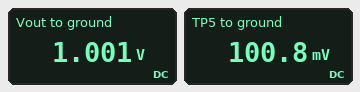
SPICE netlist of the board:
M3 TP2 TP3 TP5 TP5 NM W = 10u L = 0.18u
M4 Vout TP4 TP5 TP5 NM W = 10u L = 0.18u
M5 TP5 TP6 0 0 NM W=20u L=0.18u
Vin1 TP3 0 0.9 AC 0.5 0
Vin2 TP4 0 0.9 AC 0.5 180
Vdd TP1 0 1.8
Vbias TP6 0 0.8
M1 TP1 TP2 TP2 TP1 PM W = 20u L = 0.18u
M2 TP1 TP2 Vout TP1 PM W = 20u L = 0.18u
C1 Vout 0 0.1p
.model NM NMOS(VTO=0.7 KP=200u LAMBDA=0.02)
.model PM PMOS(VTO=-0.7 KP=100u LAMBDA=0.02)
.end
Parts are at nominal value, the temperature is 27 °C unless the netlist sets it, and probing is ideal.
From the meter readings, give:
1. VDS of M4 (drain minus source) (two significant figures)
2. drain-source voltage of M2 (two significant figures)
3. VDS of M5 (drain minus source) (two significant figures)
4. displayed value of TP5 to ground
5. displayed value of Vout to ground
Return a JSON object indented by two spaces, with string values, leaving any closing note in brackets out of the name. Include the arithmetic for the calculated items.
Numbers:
{
  "VDS of M4 (drain minus source)": "1.001 V - 100.8 mV = 900 mV",
  "drain-source voltage of M2": "1.8 V - 1.001 V = 800 mV",
  "VDS of M5 (drain minus source)": "100.8 mV = 100 mV",
  "displayed value of TP5 to ground": "100.8 mV",
  "displayed value of Vout to ground": "1.001 V"
}
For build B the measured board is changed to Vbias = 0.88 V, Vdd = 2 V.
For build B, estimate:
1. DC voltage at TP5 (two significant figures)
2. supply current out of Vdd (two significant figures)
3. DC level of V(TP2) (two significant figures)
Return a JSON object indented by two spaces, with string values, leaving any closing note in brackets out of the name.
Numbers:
{
  "DC voltage at TP5": "64 mV",
  "supply current out of Vdd": "210 µA",
  "DC level of V(TP2)": "1.2 V"
}
